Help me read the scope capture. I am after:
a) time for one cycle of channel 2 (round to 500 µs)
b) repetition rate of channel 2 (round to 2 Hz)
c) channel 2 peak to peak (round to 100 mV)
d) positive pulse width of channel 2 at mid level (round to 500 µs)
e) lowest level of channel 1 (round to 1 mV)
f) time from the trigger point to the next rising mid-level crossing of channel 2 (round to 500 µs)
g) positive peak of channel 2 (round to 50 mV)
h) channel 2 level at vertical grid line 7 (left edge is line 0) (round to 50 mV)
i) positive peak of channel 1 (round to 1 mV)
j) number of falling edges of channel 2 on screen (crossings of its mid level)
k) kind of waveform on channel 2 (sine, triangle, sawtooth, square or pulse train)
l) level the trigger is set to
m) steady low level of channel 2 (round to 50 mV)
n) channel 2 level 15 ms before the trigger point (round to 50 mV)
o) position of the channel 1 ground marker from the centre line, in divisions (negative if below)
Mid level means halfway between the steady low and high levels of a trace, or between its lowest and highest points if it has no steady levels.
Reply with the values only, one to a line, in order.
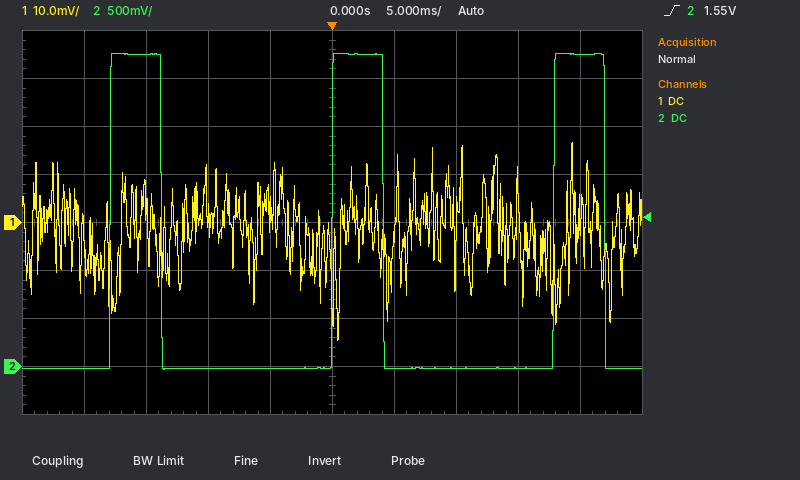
18.0 ms
56 Hz
3.30 V
4.0 ms
-25 mV
18.0 ms
3.25 V
0 mV
17 mV
3
pulse train
1.55 V
0 mV
3.25 V
0.0 div
